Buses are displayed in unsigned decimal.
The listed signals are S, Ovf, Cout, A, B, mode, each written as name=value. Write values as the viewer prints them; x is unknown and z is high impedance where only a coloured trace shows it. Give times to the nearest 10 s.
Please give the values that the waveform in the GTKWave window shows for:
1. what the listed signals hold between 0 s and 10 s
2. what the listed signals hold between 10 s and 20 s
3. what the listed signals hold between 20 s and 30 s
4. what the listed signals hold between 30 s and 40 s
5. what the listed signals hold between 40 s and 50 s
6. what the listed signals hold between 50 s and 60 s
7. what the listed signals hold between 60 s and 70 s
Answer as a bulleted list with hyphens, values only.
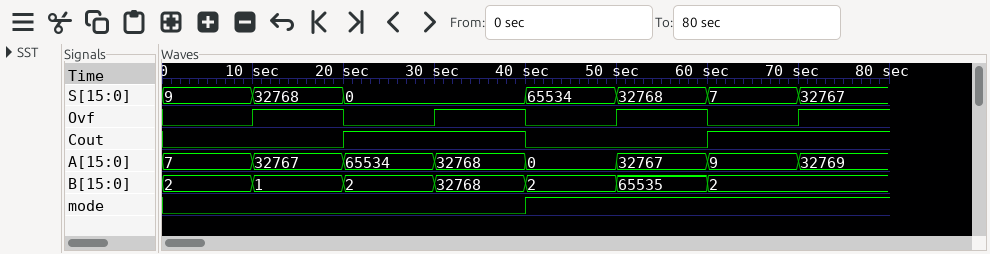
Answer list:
- S=9, Ovf=0, Cout=0, A=7, B=2, mode=0
- S=32768, Ovf=1, Cout=0, A=32767, B=1, mode=0
- S=0, Ovf=0, Cout=1, A=65534, B=2, mode=0
- S=0, Ovf=1, Cout=1, A=32768, B=32768, mode=0
- S=65534, Ovf=0, Cout=0, A=0, B=2, mode=1
- S=32768, Ovf=1, Cout=0, A=32767, B=65535, mode=1
- S=7, Ovf=0, Cout=1, A=9, B=2, mode=1
